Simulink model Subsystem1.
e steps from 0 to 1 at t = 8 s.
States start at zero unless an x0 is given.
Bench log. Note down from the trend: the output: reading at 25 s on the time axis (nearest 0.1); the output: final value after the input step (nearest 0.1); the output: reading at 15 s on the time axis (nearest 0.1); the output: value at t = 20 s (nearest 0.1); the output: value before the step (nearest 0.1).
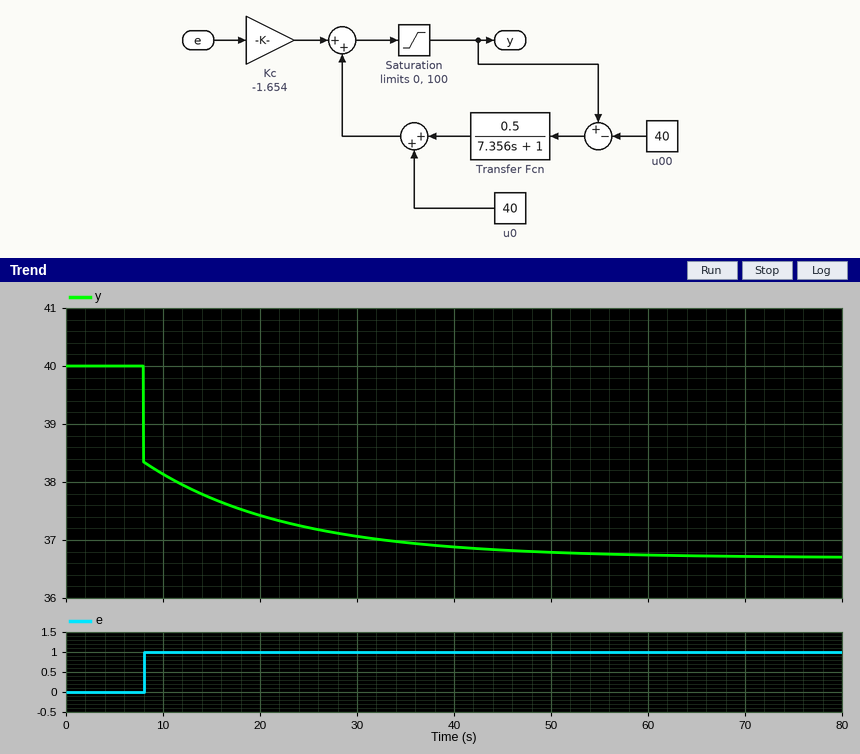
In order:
37.2
36.7
37.7
37.4
40.0
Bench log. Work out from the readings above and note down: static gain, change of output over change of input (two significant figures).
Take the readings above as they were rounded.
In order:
-3.3
